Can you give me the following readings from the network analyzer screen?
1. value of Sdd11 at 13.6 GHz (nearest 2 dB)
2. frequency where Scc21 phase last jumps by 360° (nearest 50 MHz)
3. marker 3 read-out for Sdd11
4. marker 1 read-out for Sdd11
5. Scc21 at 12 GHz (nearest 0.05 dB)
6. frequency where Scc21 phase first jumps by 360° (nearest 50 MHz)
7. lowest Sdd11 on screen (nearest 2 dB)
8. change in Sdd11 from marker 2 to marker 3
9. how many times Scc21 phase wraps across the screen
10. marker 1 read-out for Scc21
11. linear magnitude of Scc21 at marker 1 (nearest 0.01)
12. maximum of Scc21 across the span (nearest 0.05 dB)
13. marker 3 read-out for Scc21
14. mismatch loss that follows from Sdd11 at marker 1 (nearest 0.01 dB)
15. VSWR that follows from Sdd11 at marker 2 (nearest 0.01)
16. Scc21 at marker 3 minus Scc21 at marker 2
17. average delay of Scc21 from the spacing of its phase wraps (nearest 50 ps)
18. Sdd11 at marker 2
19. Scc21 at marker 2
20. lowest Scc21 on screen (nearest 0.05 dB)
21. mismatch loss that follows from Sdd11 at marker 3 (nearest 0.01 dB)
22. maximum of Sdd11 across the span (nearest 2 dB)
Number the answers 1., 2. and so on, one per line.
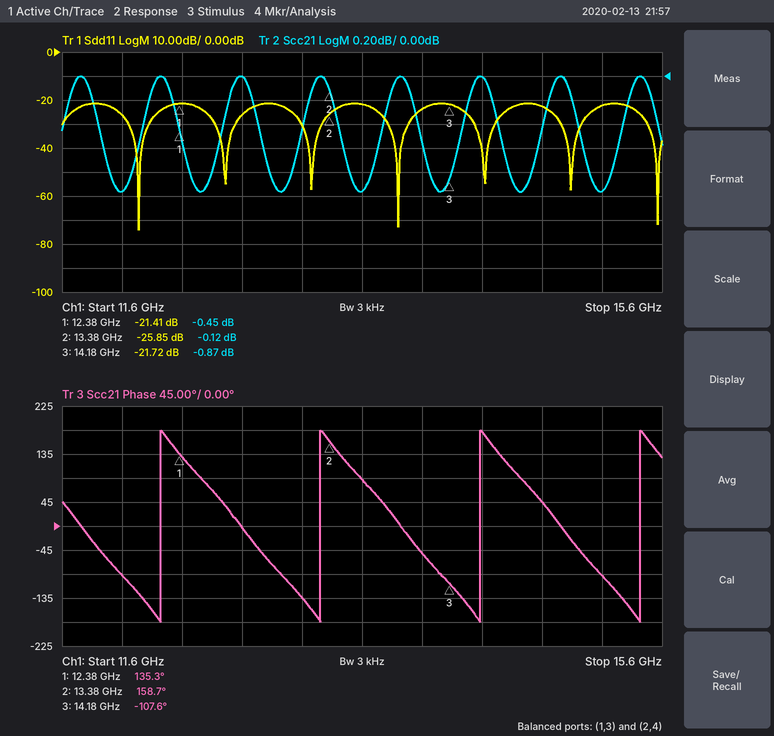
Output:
1. -22 dB
2. 15.45 GHz
3. -21.72 dB
4. -21.41 dB
5. -0.95 dB
6. 12.25 GHz
7. -74 dB
8. 4.13 dB
9. 4
10. -0.45 dB
11. 0.95
12. 0.00 dB
13. -0.87 dB
14. 0.03 dB
15. 1.11
16. -0.75 dB
17. 950 ps
18. -25.85 dB
19. -0.12 dB
20. -0.95 dB
21. 0.03 dB
22. -22 dB
